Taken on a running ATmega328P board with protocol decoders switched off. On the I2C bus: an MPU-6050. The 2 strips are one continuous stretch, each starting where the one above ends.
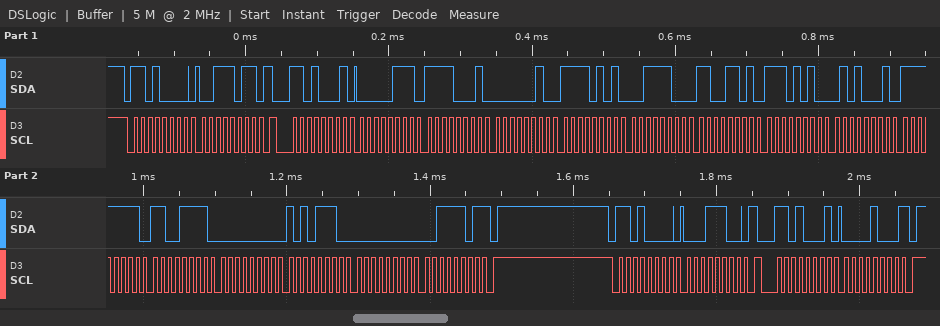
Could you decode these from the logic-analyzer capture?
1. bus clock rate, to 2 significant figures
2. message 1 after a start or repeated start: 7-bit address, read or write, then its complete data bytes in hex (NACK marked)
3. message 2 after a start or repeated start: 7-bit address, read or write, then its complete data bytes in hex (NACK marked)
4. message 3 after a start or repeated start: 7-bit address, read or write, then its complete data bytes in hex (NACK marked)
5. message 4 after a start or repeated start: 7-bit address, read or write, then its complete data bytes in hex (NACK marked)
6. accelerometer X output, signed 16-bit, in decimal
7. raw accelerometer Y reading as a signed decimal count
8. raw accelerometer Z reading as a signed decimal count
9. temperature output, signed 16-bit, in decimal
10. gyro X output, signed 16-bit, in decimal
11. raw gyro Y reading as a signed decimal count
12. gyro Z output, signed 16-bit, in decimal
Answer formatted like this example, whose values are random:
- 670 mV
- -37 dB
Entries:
- 100 kHz
- 0x68 write: 3B
- 0x68 read: 07 F1 02 F5 3C CD EA 51 FF CF 00 AE 00 3D NACK
- 0x68 write: 1C
- 0x68 read: 08 NACK
- 2033
- 757
- 15565
- -5551
- -49
- 174
- 61
